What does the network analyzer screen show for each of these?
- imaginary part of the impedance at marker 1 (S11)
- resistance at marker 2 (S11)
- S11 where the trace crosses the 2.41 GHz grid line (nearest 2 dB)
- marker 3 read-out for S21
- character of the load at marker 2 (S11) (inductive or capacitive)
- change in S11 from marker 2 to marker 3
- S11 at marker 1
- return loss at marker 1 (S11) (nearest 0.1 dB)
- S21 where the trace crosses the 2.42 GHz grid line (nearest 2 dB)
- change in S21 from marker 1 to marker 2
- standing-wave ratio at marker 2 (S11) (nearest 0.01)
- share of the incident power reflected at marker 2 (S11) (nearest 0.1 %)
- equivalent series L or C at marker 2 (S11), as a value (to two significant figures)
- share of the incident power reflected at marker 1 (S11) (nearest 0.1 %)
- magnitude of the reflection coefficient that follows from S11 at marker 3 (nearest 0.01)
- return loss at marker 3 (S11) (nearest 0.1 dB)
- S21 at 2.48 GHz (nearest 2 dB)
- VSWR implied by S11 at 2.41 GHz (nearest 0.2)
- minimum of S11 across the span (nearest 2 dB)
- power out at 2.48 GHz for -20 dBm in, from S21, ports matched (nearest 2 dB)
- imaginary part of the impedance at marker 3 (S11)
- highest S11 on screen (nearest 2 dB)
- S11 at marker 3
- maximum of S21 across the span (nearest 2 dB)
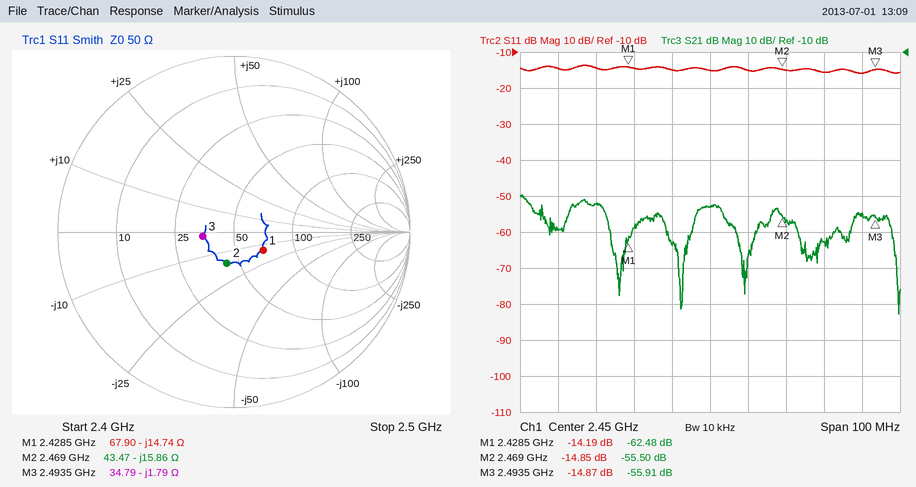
-14.74 Ω
43.47 Ω
-14 dB
-55.91 dB
capacitive
-0.02 dB
-14.19 dB
14.2 dB
-52 dB
6.98 dB
1.44
3.3 %
4.1 pF
3.8 %
0.18
14.9 dB
-62 dB
1.4
-16 dB
-82 dBm
-1.79 Ω
-14 dB
-14.87 dB
-50 dB
